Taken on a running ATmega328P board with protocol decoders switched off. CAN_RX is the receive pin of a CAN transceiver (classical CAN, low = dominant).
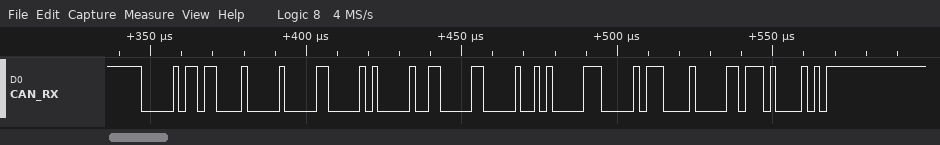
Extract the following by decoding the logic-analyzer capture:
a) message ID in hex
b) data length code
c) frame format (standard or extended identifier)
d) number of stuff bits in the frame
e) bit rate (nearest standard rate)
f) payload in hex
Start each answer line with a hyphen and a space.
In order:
- 0x036
- 8
- standard
- 10
- 500 kbit/s
- 01 02 03 04 05 06 07 08
